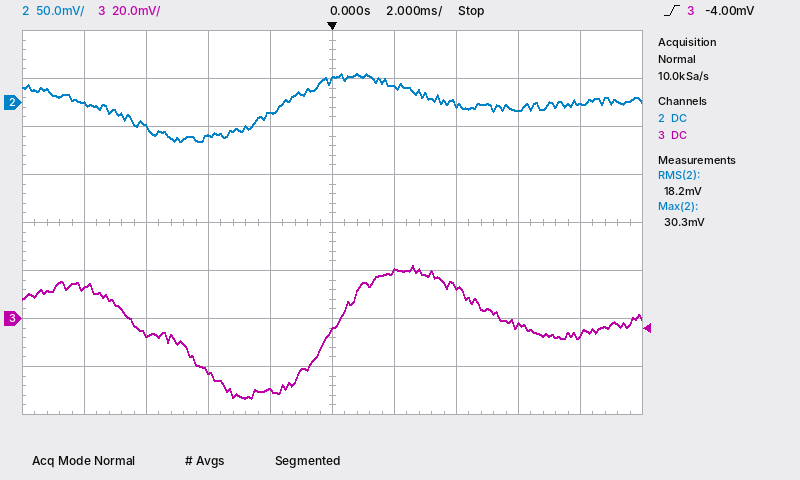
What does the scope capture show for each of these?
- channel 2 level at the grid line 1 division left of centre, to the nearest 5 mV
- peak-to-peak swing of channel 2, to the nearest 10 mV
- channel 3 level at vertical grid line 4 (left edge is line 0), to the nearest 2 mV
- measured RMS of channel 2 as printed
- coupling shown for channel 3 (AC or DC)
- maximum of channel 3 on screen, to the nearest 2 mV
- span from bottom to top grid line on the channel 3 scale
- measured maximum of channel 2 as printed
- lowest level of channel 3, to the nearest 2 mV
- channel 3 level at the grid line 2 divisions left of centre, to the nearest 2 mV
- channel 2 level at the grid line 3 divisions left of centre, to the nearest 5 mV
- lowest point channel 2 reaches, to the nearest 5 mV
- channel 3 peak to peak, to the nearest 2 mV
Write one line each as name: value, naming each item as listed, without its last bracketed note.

channel 2 level at the grid line 1 division left of centre, to the nearest 5 mV: -10 mV
peak-to-peak swing of channel 2, to the nearest 10 mV: 70 mV
channel 3 level at vertical grid line 4 (left edge is line 0), to the nearest 2 mV: -30 mV
measured RMS of channel 2 as printed: 18.2 mV
coupling shown for channel 3: DC
maximum of channel 3 on screen, to the nearest 2 mV: 22 mV
span from bottom to top grid line on the channel 3 scale: 160 mV
measured maximum of channel 2 as printed: 30.3 mV
lowest level of channel 3, to the nearest 2 mV: -34 mV
channel 3 level at the grid line 2 divisions left of centre, to the nearest 2 mV: -22 mV
channel 2 level at the grid line 3 divisions left of centre, to the nearest 5 mV: -25 mV
lowest point channel 2 reaches, to the nearest 5 mV: -40 mV
channel 3 peak to peak, to the nearest 2 mV: 56 mV
